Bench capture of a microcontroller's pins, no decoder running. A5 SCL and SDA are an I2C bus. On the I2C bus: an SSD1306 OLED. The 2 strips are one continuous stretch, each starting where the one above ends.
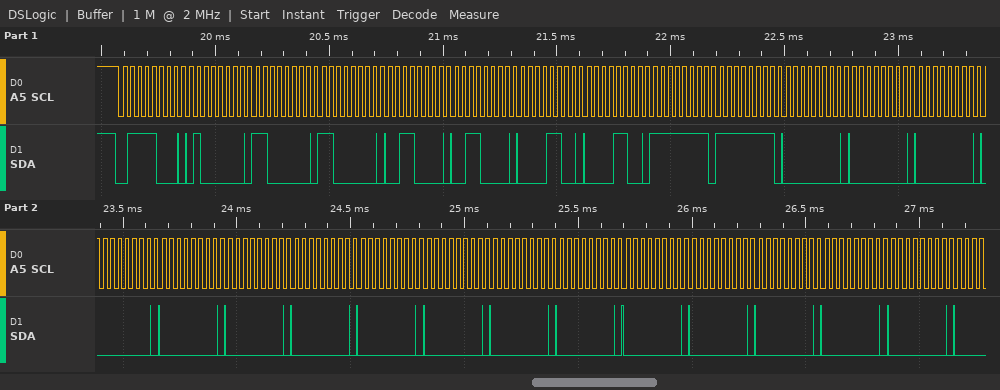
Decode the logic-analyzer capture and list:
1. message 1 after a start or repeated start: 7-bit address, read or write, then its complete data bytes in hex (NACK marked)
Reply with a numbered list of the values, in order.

1. 0x3C write: 40 C0 C0 30 30 0C 0C FF FF 00 00 00 00 00 00 00 00 00 00 00 00 00 00 00 00
